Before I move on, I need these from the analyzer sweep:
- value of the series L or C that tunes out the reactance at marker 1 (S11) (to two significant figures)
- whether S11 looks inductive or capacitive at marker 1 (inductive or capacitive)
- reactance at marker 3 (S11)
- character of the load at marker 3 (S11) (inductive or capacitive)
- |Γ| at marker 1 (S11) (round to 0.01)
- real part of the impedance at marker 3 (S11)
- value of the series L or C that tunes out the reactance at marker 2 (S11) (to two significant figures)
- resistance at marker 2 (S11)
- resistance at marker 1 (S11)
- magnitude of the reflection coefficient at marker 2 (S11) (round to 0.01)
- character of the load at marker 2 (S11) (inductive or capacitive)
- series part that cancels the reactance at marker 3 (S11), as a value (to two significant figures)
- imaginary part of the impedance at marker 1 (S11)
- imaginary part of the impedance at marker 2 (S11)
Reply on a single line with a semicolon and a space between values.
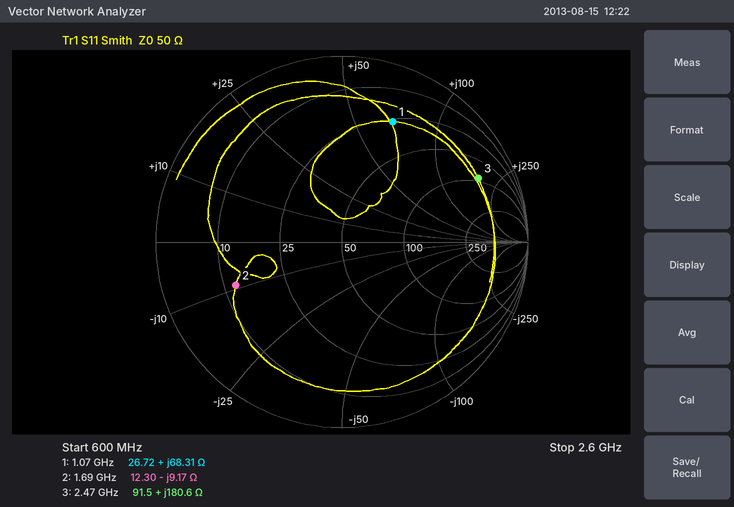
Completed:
2.2 pF; inductive; +180.6 Ω; inductive; 0.70; 91.5 Ω; 860 pH; 12.30 Ω; 26.72 Ω; 0.62; capacitive; 360 fF; +68.31 Ω; -9.17 Ω
